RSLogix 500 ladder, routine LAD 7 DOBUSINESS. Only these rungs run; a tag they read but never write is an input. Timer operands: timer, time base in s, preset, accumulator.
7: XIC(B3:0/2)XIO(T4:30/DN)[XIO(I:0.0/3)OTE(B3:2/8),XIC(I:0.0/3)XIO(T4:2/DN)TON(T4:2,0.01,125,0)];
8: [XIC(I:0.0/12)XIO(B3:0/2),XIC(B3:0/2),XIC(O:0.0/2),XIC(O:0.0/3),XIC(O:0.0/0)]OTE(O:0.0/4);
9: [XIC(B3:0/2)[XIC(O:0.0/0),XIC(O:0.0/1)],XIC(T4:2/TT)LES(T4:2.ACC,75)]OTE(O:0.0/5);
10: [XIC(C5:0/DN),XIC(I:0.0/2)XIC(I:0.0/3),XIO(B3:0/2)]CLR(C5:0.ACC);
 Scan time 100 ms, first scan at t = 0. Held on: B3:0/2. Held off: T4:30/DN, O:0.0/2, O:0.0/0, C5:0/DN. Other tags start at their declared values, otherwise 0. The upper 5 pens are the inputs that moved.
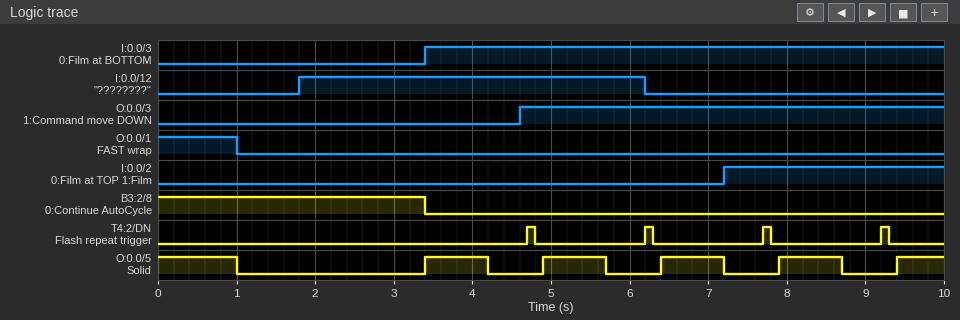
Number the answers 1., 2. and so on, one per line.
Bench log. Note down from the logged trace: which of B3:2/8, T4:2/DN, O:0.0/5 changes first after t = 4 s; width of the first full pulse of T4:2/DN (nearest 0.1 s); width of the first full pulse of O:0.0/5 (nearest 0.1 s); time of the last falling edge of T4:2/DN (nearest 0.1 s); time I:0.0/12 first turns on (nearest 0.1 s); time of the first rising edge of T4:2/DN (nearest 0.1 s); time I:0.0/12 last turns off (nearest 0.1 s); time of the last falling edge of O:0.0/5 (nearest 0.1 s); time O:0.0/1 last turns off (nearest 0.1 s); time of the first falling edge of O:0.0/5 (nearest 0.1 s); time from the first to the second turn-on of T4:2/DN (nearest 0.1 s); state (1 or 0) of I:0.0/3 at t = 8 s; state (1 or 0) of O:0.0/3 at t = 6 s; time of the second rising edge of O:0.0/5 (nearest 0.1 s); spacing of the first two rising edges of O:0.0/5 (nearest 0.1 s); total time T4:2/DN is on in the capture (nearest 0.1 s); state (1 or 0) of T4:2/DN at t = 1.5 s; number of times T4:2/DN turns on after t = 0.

1. O:0.0/5
2. 0.1 s
3. 0.8 s
4. 9.3 s
5. 1.8 s
6. 4.7 s
7. 6.2 s
8. 8.7 s
9. 1.0 s
10. 1.0 s
11. 1.5 s
12. 1
13. 1
14. 4.9 s
15. 1.5 s
16. 0.4 s
17. 0
18. 4
